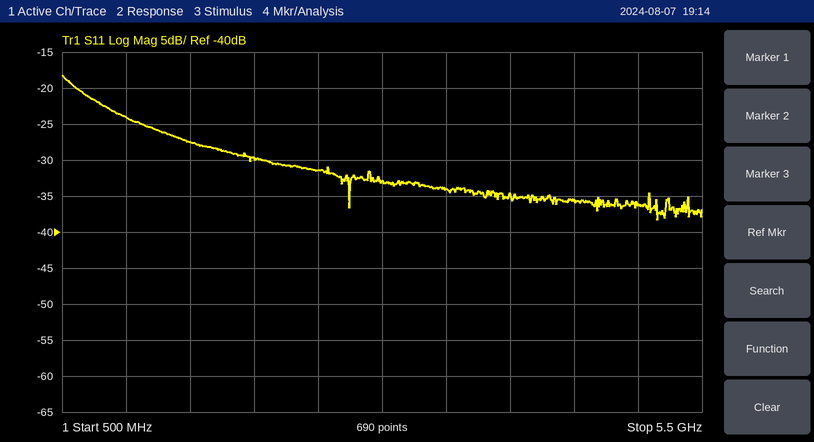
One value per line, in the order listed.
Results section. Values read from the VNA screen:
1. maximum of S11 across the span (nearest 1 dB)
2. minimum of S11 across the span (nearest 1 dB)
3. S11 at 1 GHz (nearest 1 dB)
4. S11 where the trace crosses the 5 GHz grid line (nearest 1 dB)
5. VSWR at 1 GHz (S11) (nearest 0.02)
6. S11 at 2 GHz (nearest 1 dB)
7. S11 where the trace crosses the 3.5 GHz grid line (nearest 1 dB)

-18 dB
-38 dB
-24 dB
-36 dB
1.14
-30 dB
-34 dB
